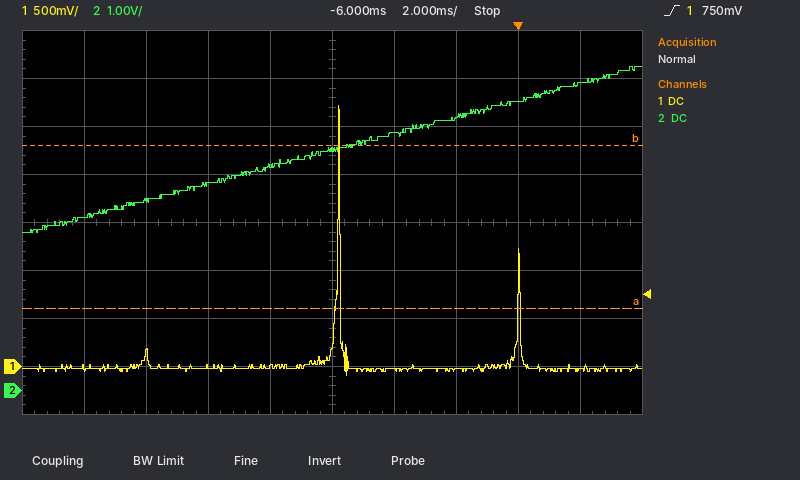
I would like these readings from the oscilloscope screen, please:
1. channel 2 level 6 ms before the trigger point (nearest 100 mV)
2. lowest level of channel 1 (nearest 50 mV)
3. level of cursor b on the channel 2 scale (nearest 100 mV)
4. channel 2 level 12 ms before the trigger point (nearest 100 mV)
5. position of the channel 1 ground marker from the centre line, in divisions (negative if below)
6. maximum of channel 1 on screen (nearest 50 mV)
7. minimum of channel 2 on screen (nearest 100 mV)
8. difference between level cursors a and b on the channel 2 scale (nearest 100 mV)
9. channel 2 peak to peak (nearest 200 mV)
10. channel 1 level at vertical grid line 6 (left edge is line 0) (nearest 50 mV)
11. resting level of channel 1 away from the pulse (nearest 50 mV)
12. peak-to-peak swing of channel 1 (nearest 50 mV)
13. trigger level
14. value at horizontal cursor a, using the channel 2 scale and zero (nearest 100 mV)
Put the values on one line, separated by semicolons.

5.0 V; -100 mV; 5.1 V; 4.0 V; -3.0 div; 2.70 V; 3.3 V; 3.4 V; 3.4 V; -50 mV; 0 mV; 2.80 V; 750 mV; 1.7 V
